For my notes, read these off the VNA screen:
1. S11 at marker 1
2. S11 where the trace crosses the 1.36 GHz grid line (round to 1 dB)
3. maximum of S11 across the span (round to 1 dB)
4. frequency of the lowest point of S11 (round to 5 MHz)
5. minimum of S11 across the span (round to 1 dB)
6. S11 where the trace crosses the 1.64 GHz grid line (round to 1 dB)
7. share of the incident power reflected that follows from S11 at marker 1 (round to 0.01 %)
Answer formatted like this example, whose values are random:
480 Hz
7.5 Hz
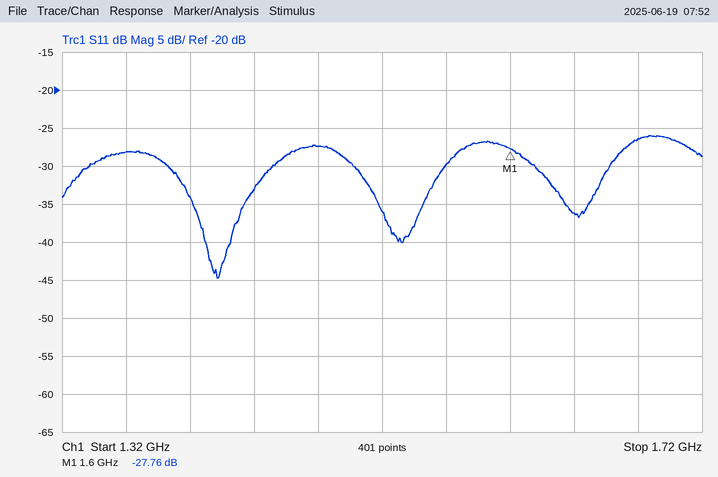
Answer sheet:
-27.76 dB
-28 dB
-26 dB
1.415 GHz
-45 dB
-36 dB
0.17 %
